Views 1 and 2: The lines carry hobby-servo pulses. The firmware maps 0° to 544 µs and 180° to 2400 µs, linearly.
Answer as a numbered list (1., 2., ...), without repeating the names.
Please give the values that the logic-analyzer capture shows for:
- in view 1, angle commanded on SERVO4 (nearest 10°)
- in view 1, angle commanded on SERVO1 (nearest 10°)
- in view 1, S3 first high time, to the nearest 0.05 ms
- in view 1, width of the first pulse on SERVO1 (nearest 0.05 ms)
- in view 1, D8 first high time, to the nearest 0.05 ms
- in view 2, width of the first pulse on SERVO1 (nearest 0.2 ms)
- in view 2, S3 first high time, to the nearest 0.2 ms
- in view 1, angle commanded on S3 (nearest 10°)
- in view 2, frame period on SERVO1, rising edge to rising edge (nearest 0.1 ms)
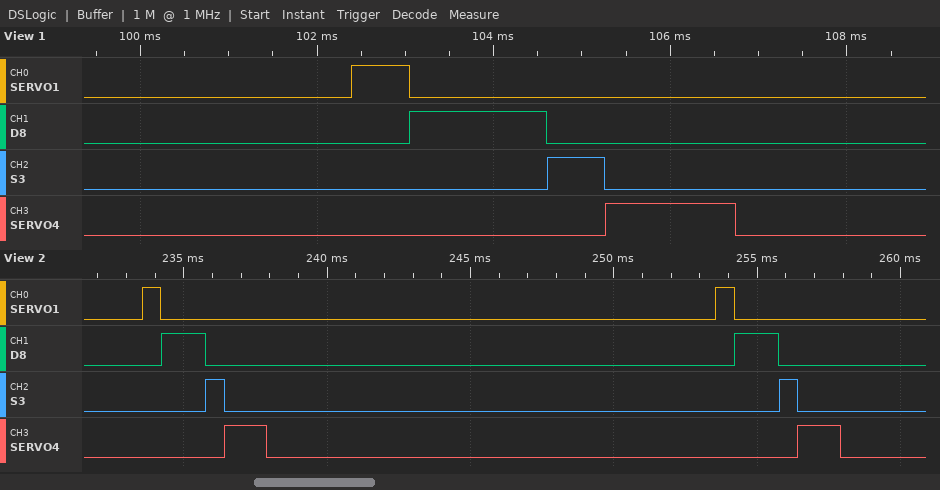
1. 90°
2. 10°
3. 0.65 ms
4. 0.65 ms
5. 1.55 ms
6. 0.6 ms
7. 0.6 ms
8. 10°
9. 20.0 ms
